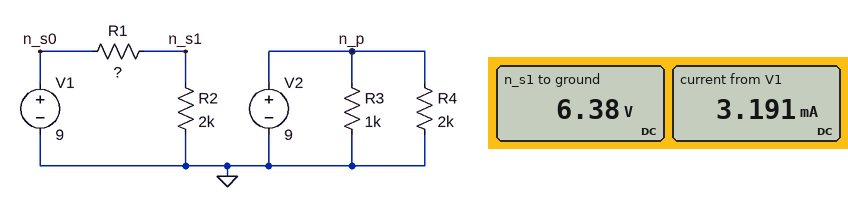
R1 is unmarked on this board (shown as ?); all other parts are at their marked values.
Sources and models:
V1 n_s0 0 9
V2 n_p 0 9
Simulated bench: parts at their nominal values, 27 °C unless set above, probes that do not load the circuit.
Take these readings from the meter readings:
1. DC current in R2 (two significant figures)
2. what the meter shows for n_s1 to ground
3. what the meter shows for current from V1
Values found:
3.2 mA
6.38 V
3.191 mA
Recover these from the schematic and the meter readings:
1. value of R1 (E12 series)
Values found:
820 Ω
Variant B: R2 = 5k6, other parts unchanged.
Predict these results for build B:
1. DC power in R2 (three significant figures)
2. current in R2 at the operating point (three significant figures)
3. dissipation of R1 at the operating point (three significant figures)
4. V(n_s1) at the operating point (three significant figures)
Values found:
11.0 mW
1.40 mA
1.61 mW
7.85 V
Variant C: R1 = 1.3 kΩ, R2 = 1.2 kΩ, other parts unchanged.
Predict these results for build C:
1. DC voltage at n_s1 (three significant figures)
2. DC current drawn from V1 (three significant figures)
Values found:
4.32 V
3.60 mA
